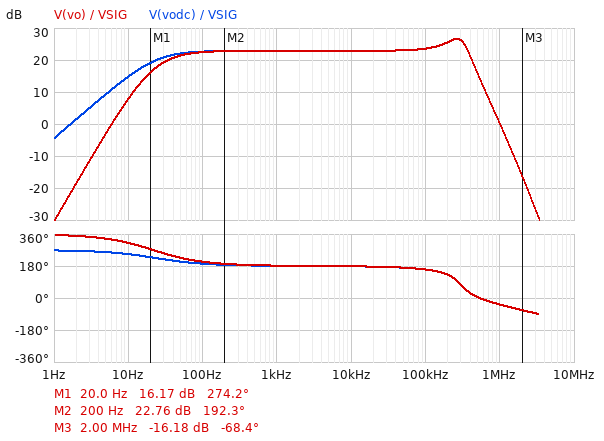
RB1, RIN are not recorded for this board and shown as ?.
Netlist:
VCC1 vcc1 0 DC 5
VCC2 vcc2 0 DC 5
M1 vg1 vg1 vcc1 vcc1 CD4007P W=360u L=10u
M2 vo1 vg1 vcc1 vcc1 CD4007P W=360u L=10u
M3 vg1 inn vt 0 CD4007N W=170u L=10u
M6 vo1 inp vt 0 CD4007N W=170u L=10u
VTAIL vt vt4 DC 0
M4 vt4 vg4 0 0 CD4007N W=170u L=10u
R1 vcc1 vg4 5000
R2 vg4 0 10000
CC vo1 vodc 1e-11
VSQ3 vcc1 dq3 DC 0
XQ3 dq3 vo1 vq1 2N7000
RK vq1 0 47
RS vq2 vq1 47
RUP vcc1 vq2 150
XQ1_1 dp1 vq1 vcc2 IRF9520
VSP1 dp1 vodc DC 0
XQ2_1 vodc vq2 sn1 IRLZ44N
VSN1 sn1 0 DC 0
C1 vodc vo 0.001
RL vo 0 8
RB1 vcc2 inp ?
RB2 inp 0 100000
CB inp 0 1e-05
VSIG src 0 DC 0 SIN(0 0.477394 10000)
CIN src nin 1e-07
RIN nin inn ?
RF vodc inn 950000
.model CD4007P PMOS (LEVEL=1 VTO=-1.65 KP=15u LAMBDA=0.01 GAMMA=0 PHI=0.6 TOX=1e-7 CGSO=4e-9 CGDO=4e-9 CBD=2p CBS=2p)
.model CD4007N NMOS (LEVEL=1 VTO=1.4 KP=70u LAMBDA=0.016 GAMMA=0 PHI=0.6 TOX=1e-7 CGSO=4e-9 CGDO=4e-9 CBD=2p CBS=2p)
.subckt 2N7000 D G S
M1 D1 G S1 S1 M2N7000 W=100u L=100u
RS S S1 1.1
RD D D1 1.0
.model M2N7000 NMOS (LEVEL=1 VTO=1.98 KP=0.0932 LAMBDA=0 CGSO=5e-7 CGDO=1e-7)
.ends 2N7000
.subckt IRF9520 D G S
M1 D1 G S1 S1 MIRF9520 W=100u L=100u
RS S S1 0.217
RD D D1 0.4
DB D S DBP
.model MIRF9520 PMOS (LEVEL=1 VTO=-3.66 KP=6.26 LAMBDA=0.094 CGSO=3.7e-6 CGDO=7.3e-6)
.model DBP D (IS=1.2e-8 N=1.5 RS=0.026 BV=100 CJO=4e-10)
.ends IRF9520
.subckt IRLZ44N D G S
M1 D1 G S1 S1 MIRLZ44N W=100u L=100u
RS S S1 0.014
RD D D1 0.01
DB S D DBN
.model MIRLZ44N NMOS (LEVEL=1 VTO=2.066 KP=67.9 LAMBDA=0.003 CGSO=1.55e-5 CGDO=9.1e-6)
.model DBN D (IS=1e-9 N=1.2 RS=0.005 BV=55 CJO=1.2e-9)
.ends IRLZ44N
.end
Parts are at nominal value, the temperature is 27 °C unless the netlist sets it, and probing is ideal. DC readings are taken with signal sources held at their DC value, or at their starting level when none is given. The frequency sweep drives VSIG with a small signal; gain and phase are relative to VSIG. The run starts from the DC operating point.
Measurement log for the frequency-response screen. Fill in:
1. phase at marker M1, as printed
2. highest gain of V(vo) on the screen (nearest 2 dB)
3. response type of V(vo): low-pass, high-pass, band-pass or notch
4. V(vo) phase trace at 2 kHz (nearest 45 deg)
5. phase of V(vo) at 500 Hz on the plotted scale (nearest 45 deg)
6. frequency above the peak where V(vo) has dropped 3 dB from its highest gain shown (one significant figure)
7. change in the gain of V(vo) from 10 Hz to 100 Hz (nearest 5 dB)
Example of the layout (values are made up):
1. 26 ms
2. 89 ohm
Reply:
1. 274.2 deg
2. 26 dB
3. band-pass
4. 180 deg
5. 180 deg
6. 400 kHz
7. 15 dB
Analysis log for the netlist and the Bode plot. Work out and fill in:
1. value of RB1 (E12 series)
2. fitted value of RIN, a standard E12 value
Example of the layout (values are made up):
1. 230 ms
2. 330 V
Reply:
1. 180 kΩ
2. 68 kΩ
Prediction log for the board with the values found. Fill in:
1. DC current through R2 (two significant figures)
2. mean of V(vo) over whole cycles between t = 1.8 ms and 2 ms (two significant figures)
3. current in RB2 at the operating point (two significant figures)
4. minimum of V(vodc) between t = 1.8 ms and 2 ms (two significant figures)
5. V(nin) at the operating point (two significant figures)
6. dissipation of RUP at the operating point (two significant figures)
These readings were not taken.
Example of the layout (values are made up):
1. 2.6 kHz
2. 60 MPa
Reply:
1. 330 µA
2. 270 mV
3. 18 µA
4. 10 mV
5. 1.8 V
6. 56 mW
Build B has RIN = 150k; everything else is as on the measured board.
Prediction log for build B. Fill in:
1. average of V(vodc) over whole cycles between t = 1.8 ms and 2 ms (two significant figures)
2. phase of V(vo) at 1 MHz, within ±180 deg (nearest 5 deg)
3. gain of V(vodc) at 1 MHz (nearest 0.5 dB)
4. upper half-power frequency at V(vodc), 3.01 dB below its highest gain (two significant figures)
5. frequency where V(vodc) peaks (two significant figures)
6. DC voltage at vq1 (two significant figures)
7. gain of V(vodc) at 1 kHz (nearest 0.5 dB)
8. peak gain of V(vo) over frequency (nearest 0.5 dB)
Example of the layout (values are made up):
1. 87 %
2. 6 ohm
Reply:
1. 2.0 V
2. -55 deg
3. -4.5 dB
4. 380 kHz
5. 360 kHz
6. 1.2 V
7. 16.0 dB
8. 37.5 dB
